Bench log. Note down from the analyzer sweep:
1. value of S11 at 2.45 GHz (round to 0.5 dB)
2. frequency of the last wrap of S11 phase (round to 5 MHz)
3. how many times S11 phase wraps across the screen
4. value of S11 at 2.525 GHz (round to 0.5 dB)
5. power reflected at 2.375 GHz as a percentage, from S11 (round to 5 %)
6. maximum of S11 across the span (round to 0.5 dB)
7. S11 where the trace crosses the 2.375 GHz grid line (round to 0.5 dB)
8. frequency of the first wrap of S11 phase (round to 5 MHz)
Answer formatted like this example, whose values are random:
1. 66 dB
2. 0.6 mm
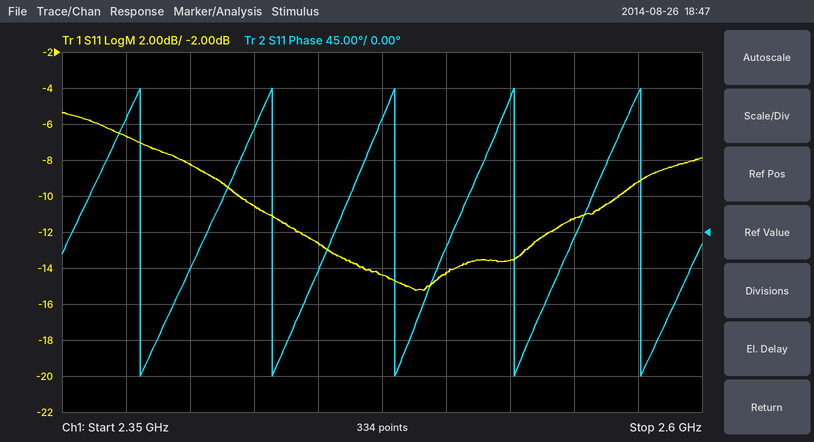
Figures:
1. -12.5 dB
2. 2.575 GHz
3. 5
4. -13.5 dB
5. 20 %
6. -5.5 dB
7. -6.5 dB
8. 2.380 GHz
